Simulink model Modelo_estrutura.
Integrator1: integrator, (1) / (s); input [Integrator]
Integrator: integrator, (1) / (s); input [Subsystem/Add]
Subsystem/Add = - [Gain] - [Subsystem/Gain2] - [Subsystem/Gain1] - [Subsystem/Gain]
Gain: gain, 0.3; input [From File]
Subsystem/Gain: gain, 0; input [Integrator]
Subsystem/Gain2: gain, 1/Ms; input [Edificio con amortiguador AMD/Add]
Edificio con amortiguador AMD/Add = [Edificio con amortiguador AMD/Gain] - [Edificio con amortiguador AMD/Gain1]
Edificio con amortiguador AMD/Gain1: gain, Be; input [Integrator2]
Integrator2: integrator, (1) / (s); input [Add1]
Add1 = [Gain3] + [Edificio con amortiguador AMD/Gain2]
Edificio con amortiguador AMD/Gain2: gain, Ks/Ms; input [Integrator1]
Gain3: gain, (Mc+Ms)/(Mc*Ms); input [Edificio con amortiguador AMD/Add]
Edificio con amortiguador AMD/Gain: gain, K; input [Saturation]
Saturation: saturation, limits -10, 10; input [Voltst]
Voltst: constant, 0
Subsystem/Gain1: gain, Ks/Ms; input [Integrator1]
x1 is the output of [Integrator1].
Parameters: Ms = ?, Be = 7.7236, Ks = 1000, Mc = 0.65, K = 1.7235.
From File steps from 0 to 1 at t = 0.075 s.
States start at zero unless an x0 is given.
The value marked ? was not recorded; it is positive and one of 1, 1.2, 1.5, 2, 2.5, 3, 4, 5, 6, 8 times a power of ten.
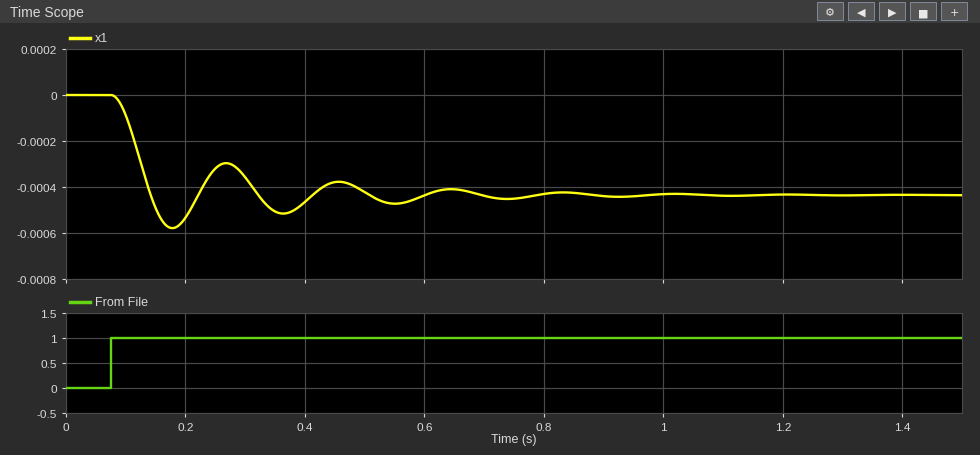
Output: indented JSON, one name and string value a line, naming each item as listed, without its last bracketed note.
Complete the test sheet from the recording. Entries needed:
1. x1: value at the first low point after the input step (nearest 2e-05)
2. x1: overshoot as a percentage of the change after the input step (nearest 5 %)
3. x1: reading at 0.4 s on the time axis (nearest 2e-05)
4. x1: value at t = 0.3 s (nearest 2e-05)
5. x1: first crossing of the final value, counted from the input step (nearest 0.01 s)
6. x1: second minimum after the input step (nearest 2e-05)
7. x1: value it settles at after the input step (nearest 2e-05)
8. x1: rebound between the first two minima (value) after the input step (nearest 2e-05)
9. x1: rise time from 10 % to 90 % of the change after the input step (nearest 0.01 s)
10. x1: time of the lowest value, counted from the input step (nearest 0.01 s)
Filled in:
{
  "x1: value at the first low point after the input step": "-0.00058",
  "x1: overshoot as a percentage of the change after the input step": "35 %",
  "x1: reading at 0.4 s on the time axis": "-0.00046",
  "x1: value at t = 0.3 s": "-0.00036",
  "x1: first crossing of the final value, counted from the input step": "0.07 s",
  "x1: second minimum after the input step": "-0.00052",
  "x1: value it settles at after the input step": "-0.00044",
  "x1: rebound between the first two minima (value) after the input step": "-0.00030",
  "x1: rise time from 10 % to 90 % of the change after the input step": "0.04 s",
  "x1: time of the lowest value, counted from the input step": "0.10 s"
}
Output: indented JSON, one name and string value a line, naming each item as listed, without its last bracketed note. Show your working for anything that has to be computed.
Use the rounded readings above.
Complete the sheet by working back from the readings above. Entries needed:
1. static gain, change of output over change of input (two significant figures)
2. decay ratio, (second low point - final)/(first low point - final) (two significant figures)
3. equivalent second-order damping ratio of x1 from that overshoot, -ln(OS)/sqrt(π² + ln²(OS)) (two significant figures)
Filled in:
{
  "static gain, change of output over change of input": "(-0.00044 - 0) / (1 - 0) = -0.00044",
  "decay ratio, (second low point - final)/(first low point - final)": "(-0.00052 - (-0.00044)) / (-0.00058 - (-0.00044)) = 0.57",
  "equivalent second-order damping ratio of x1 from that overshoot, -ln(OS)/sqrt(π² + ln²(OS))": "ln(0.35) = -1.050; 1.050 / sqrt(9.870 + 1.102) = 0.32"
}
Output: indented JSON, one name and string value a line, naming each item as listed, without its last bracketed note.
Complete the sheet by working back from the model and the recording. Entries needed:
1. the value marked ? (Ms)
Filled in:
{
  "the value marked ?": "0.8"
}
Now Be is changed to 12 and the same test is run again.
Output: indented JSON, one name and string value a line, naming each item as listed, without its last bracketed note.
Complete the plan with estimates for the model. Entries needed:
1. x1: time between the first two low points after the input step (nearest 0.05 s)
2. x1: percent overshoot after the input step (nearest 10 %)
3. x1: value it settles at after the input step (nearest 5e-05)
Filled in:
{
  "x1: time between the first two low points after the input step": "0.20 s",
  "x1: percent overshoot after the input step": "40 %",
  "x1: value it settles at after the input step": "-0.00045"
}
